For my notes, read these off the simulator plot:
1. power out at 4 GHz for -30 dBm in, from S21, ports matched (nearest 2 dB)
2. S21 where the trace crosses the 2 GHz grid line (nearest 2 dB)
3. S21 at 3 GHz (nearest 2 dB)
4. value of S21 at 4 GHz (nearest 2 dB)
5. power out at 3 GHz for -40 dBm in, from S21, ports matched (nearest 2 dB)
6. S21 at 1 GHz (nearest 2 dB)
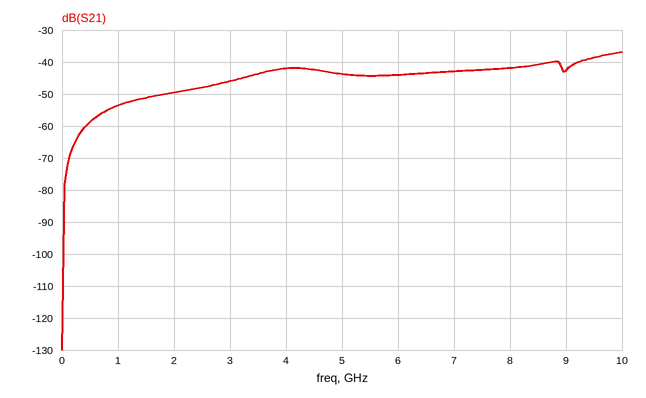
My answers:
-72 dBm
-50 dB
-46 dB
-42 dB
-86 dBm
-54 dB
